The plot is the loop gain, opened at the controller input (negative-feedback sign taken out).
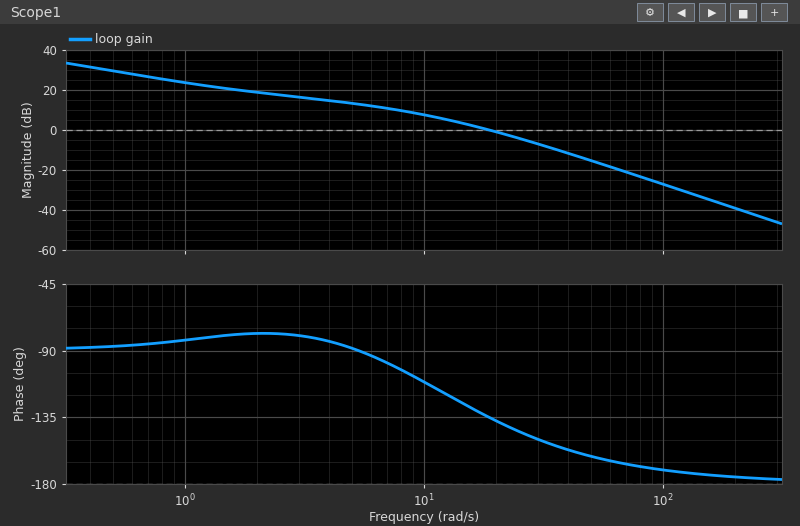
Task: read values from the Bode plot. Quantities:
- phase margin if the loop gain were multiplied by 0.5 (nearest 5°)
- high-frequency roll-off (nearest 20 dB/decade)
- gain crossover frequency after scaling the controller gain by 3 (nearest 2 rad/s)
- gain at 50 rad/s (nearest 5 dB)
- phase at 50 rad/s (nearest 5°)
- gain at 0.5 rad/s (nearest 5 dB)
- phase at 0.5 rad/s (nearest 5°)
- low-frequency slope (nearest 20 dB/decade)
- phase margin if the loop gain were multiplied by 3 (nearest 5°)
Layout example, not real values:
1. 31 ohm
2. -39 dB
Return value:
1. 65°
2. -40 dB/decade
3. 36 rad/s
4. -15 dB
5. -160°
6. 30 dB
7. -85°
8. -20 dB/decade
9. 25°
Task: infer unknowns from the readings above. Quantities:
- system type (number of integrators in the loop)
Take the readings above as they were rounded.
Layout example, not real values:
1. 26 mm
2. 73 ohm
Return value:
1. 1
